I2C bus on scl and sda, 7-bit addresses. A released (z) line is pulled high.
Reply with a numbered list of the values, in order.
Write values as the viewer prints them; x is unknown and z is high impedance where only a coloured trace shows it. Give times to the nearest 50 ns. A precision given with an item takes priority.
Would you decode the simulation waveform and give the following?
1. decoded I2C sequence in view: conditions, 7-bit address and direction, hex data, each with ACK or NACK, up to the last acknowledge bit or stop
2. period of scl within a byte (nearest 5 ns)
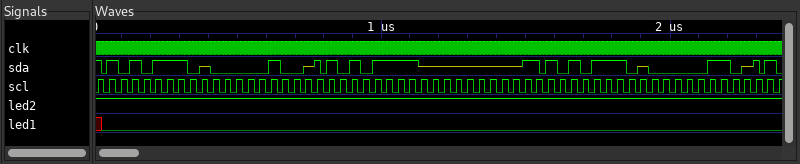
1. start, address 57 write NACK, 04 NACK, repeated start, address 57 read NACK, FF NACK, repeated start, address 57 write NACK, 06 NACK
2. 40 ns
